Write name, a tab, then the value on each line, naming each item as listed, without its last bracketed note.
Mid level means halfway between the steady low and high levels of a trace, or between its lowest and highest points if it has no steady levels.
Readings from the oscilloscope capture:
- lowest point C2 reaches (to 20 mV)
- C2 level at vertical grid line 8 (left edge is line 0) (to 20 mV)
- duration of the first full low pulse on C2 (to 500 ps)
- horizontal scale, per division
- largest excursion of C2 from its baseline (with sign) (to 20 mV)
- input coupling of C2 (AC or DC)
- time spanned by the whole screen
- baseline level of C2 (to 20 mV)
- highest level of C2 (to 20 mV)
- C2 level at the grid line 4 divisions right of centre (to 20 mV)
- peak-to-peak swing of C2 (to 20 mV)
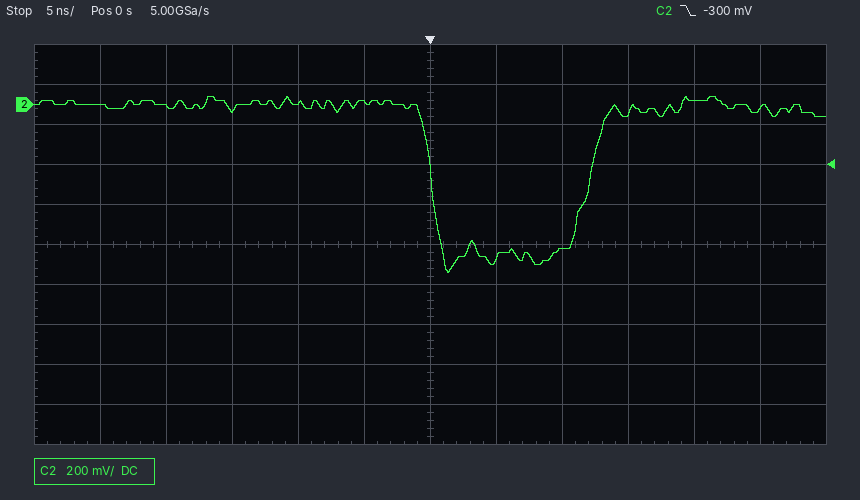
lowest point C2 reaches	-840 mV
C2 level at vertical grid line 8 (left edge is line 0)	-720 mV
duration of the first full low pulse on C2	12.0 ns
horizontal scale, per division	5 ns
largest excursion of C2 from its baseline (with sign)	-840 mV
input coupling of C2	DC
time spanned by the whole screen	60 ns
baseline level of C2	0 mV
highest level of C2	40 mV
C2 level at the grid line 4 divisions right of centre	20 mV
peak-to-peak swing of C2	880 mV
